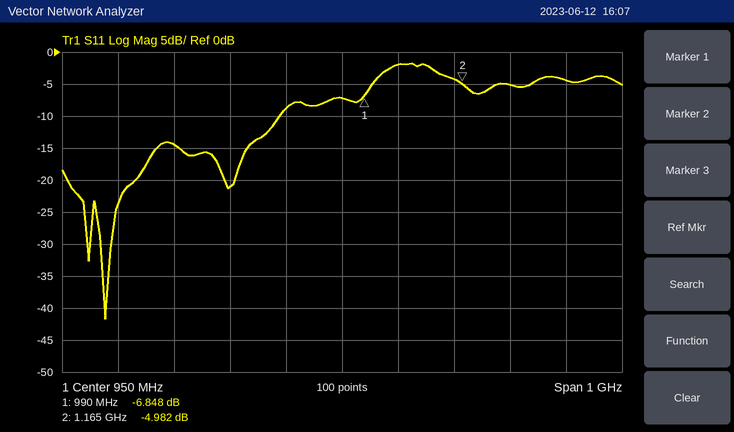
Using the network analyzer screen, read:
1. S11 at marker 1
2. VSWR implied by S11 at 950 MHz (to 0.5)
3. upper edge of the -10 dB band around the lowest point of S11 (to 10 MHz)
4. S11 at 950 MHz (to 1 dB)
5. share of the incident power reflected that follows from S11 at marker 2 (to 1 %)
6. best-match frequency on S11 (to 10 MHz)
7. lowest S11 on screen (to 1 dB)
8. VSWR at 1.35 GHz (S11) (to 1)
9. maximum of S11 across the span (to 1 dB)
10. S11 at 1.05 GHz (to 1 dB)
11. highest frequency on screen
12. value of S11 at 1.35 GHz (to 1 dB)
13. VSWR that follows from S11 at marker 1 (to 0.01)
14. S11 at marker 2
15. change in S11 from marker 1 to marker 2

-6.848 dB
2.5
840 MHz
-7 dB
32 %
530 MHz
-42 dB
4
-2 dB
-2 dB
1.45 GHz
-4 dB
2.67
-4.982 dB
1.866 dB
